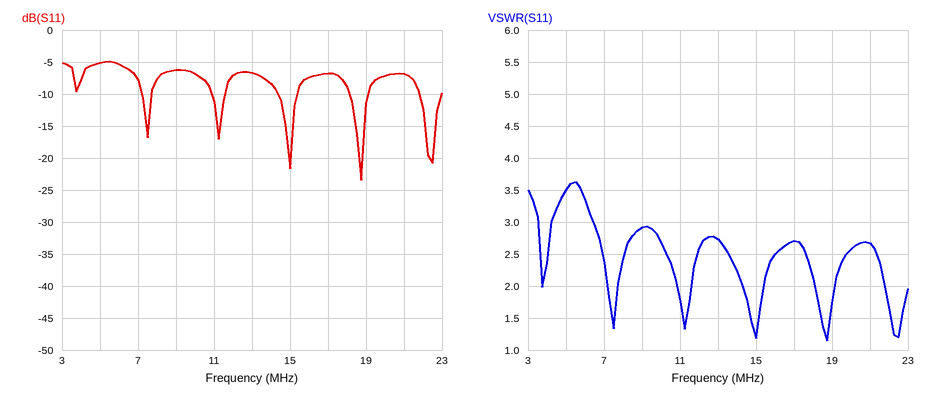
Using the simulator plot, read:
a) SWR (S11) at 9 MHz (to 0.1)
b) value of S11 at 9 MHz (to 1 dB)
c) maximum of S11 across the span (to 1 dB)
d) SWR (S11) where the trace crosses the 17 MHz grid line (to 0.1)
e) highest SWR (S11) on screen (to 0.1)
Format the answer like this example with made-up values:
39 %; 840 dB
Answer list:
2.9; -6 dB; -5 dB; 2.7; 3.6
